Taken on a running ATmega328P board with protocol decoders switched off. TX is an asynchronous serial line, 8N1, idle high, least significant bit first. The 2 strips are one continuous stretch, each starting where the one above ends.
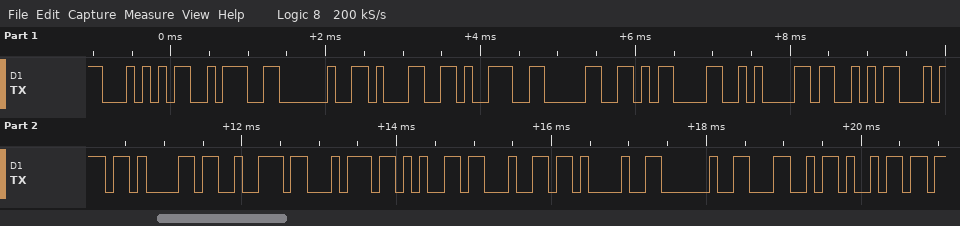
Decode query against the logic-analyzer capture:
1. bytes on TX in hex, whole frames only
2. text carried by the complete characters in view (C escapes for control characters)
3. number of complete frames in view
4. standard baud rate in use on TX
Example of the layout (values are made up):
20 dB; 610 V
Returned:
0x54 0x3A 0x20 0x31 0x39 0x30 0x0D 0x0A 0x53 0x74 0x61 0x72 0x74 0x65 0x64 0x21 0x20 0x4C 0x69; "T: 190\r\nStarted! Li"; 19; 9600 baud
